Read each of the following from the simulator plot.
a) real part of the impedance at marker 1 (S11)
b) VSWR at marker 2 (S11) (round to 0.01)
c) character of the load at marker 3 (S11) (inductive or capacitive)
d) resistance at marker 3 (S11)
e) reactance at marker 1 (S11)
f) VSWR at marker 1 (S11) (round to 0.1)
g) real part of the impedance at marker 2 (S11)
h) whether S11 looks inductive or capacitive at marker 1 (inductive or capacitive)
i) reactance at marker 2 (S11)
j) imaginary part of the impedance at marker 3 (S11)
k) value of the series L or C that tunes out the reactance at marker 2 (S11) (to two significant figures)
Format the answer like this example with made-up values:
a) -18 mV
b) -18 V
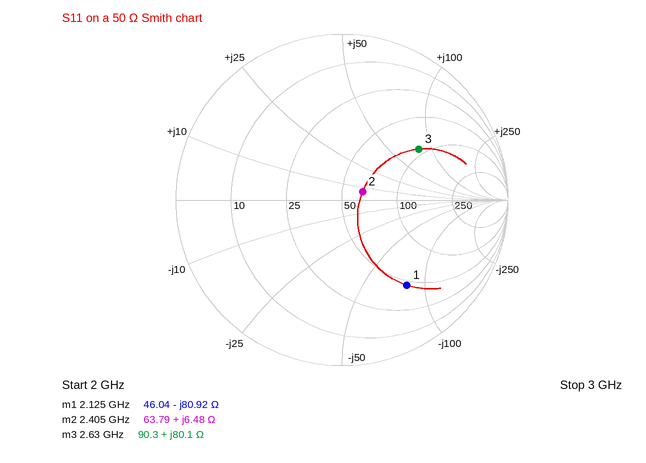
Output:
a) 46.04 Ω
b) 1.31
c) inductive
d) 90.3 Ω
e) -80.92 Ω
f) 4.6
g) 63.79 Ω
h) capacitive
i) +6.48 Ω
j) +80.1 Ω
k) 10 pF
